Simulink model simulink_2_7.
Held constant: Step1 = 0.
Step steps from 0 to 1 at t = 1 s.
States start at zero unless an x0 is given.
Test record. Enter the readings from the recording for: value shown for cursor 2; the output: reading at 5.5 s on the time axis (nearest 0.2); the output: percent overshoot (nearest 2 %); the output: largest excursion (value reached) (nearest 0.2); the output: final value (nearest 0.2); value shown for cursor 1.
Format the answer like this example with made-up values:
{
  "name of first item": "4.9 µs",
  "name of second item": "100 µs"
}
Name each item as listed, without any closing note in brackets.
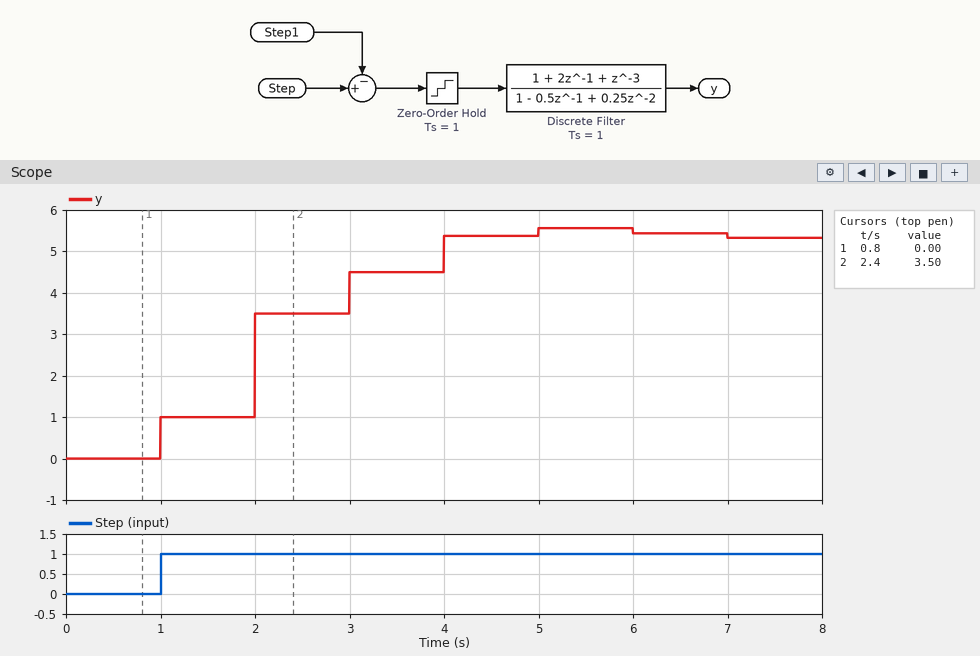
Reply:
{
  "value shown for cursor 2": "3.50",
  "the output: reading at 5.5 s on the time axis": "5.6",
  "the output: percent overshoot": "4 %",
  "the output: largest excursion (value reached)": "5.6",
  "the output: final value": "5.4",
  "value shown for cursor 1": "0.00"
}
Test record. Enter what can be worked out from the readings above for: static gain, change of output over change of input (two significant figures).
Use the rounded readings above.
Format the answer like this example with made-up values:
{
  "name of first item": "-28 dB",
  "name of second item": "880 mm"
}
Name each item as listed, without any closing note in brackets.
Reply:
{
  "static gain, change of output over change of input": "5.4"
}
